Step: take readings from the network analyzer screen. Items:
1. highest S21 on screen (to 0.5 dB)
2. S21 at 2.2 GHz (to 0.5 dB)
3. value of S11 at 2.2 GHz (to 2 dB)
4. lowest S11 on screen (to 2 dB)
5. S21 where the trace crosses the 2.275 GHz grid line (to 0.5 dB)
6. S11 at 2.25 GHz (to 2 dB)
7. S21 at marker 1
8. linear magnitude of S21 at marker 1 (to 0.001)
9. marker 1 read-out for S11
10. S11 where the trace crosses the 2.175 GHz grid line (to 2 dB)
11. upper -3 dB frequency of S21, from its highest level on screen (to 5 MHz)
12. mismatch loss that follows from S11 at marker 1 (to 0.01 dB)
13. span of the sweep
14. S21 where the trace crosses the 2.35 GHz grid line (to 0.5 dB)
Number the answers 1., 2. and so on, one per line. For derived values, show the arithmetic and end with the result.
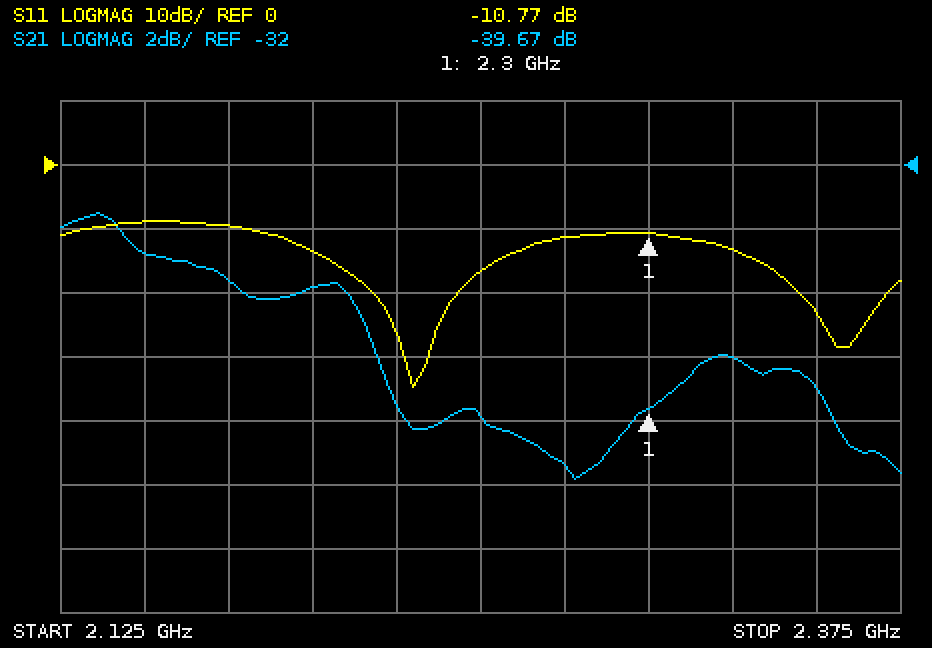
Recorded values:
1. -33.5 dB
2. -36.0 dB
3. -14 dB
4. -34 dB
5. -41.5 dB
6. -16 dB
7. -39.67 dB
8. 10^(-39.67/20) ≈ 0.010
9. -10.77 dB
10. -10 dB
11. 2.215 GHz
12. −10 log10(1 − 10^(-10.77/10)) ≈ 0.38 dB
13. 250 MHz
14. -39.0 dB
